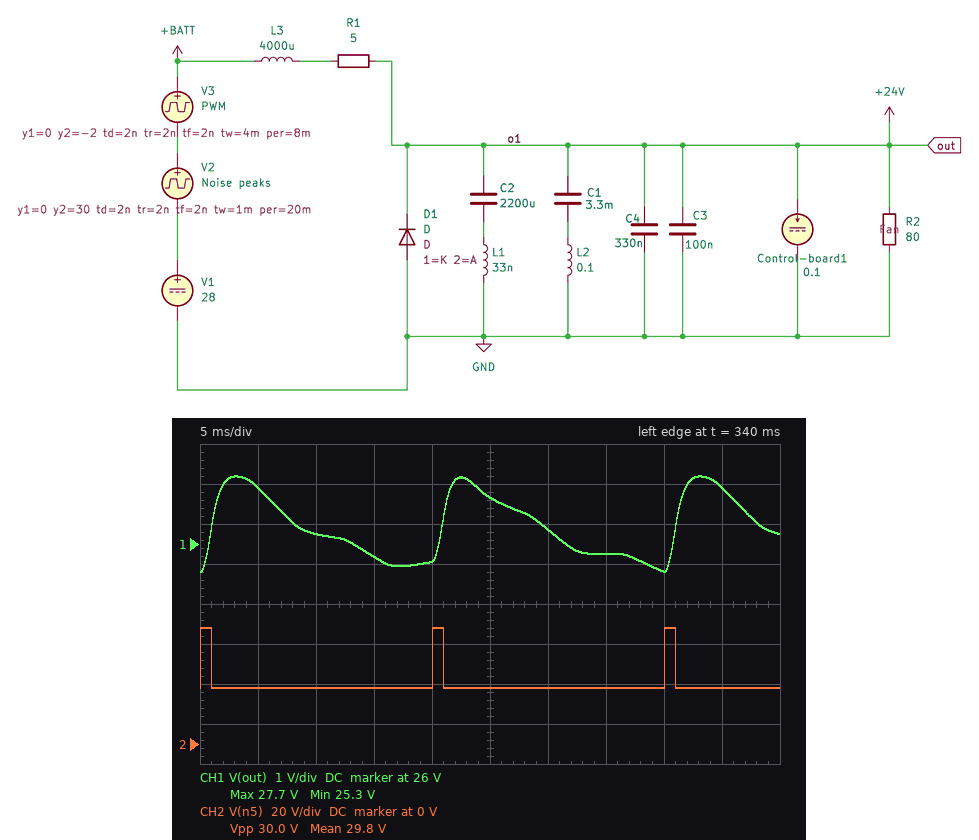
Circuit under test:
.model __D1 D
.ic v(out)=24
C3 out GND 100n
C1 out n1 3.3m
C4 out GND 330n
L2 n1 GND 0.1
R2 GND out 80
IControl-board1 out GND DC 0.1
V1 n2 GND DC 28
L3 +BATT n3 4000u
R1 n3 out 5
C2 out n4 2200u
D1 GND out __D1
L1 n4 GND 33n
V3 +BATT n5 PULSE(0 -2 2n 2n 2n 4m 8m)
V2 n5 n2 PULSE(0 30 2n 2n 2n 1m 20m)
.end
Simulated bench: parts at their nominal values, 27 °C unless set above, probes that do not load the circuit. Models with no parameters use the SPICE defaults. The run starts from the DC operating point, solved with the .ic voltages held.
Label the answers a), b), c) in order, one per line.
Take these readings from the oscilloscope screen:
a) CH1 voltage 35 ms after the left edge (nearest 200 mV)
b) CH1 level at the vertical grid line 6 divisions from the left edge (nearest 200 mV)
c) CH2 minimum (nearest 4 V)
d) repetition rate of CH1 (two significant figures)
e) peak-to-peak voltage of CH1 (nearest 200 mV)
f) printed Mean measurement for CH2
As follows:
a) 25.8 V
b) 26.4 V
c) 28 V
d) 50 Hz
e) 2.4 V
f) 29.8 V
